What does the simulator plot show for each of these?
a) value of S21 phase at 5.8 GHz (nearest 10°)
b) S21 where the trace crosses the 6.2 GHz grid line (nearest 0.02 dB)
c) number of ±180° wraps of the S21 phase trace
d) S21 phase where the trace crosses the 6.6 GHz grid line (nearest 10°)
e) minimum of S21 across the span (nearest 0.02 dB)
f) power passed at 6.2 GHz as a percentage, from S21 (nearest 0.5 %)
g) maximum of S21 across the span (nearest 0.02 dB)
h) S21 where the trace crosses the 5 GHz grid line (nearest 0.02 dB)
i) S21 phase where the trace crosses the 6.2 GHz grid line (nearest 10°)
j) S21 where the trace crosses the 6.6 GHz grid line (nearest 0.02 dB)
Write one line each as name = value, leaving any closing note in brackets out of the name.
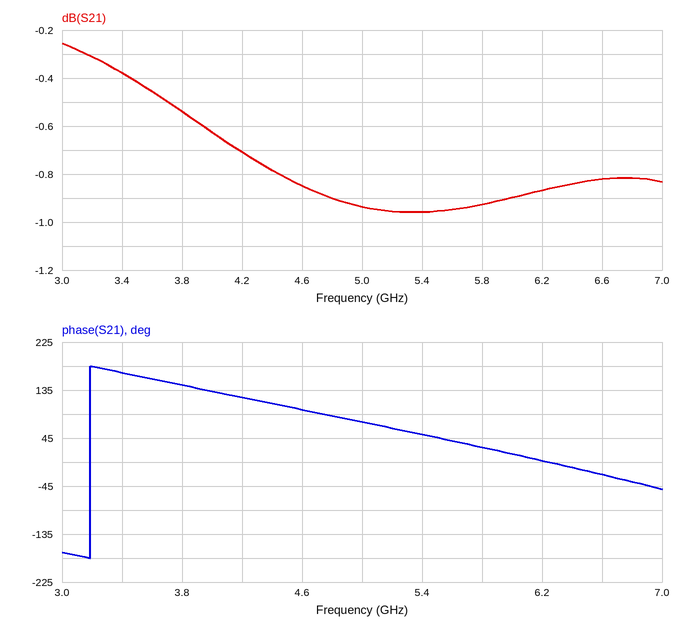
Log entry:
value of S21 phase at 5.8 GHz = 30°
S21 where the trace crosses the 6.2 GHz grid line = -0.86 dB
number of ±180° wraps of the S21 phase trace = 1
S21 phase where the trace crosses the 6.6 GHz grid line = -20°
minimum of S21 across the span = -0.96 dB
power passed at 6.2 GHz as a percentage, from S21 = 82.0 %
maximum of S21 across the span = -0.26 dB
S21 where the trace crosses the 5 GHz grid line = -0.94 dB
S21 phase where the trace crosses the 6.2 GHz grid line = 0°
S21 where the trace crosses the 6.6 GHz grid line = -0.82 dB
